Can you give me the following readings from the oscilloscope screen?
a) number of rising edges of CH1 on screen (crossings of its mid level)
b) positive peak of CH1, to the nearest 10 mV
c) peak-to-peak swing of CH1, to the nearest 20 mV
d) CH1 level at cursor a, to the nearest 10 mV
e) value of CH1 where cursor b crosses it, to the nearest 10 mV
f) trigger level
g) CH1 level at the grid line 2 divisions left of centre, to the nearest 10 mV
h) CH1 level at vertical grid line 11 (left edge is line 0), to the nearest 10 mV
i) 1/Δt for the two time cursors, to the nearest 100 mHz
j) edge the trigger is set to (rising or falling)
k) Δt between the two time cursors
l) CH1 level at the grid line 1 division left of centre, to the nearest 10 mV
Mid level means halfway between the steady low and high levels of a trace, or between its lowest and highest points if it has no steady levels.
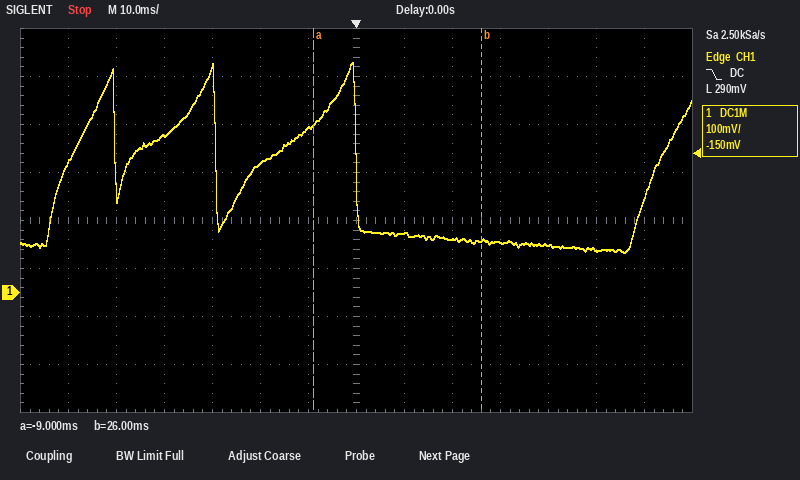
4
480 mV
400 mV
350 mV
110 mV
290 mV
270 mV
100 mV
28.6 Hz
falling
35 ms
340 mV
